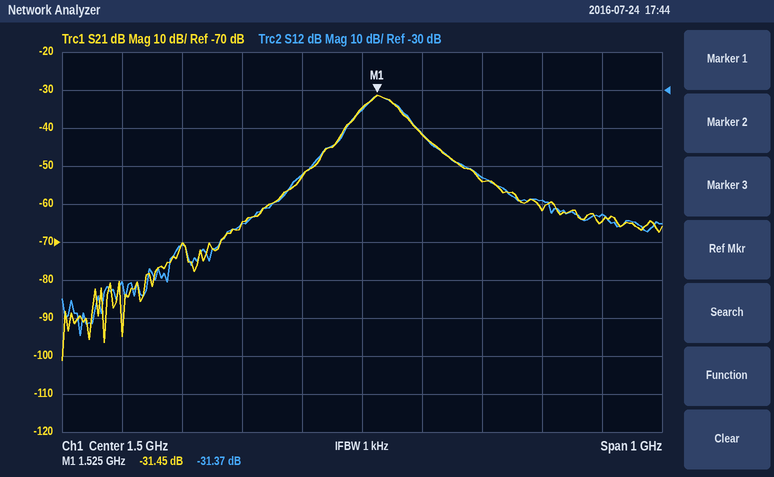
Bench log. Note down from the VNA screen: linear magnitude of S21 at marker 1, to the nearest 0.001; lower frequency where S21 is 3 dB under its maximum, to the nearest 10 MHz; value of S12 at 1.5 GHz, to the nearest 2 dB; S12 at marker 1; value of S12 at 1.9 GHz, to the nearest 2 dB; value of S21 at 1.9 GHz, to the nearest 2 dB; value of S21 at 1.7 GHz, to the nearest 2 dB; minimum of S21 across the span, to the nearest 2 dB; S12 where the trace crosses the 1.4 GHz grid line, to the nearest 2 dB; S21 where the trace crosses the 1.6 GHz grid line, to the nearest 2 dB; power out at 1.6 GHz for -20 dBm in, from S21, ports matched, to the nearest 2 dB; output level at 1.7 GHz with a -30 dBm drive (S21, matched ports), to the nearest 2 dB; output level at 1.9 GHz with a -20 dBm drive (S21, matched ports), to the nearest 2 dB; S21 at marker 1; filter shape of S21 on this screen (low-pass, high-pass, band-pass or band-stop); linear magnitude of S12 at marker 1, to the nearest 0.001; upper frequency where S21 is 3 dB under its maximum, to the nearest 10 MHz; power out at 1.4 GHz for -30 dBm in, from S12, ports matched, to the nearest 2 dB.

0.027
1.50 GHz
-36 dB
-31.37 dB
-62 dB
-64 dB
-54 dB
-102 dB
-52 dB
-42 dB
-62 dBm
-84 dBm
-84 dBm
-31.45 dB
band-pass
0.027
1.56 GHz
-82 dBm
